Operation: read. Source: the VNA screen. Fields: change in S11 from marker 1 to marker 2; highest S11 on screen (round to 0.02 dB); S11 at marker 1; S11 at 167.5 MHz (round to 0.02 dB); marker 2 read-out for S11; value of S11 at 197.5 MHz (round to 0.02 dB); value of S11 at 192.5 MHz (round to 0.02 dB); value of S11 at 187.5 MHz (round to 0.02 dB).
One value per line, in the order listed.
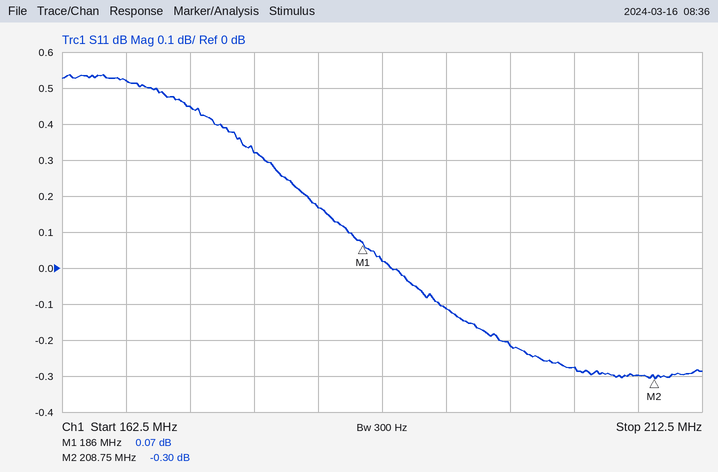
-0.37 dB
0.54 dB
0.07 dB
0.52 dB
-0.30 dB
-0.22 dB
-0.12 dB
0.02 dB
